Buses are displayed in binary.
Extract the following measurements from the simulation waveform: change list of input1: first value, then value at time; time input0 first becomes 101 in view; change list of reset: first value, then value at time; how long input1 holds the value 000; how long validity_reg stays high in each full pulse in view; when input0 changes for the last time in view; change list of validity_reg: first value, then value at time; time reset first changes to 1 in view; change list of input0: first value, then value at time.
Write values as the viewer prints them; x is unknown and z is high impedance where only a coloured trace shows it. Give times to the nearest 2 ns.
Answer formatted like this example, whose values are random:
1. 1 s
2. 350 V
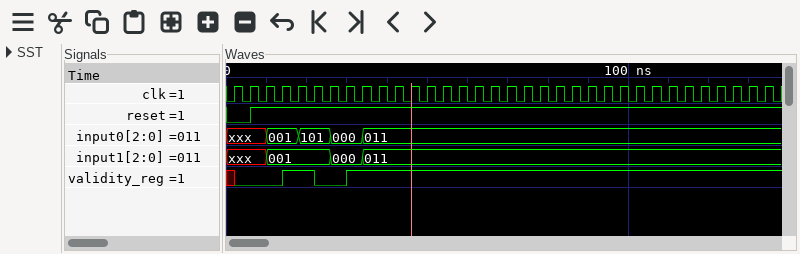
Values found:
1. xxx, 001 at 10 ns, 000 at 26 ns, 011 at 34 ns
2. 18 ns
3. 0, 1 at 6 ns
4. 8 ns
5. 8 ns
6. 34 ns
7. x, 0 at 2 ns, 1 at 14 ns, 0 at 22 ns, 1 at 30 ns
8. 6 ns
9. xxx, 001 at 10 ns, 101 at 18 ns, 000 at 26 ns, 011 at 34 ns
